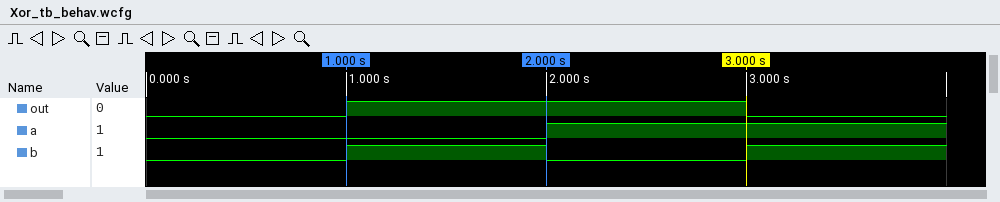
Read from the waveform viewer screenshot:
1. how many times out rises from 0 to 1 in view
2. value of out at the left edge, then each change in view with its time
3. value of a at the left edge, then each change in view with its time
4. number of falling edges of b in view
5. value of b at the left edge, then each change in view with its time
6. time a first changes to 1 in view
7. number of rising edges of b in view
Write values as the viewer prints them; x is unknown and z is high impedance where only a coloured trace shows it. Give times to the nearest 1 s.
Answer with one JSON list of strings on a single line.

["1", "0, 1 at 1 s, 0 at 3 s", "0, 1 at 2 s", "1", "0, 1 at 1 s, 0 at 2 s, 1 at 3 s", "2 s", "2"]
